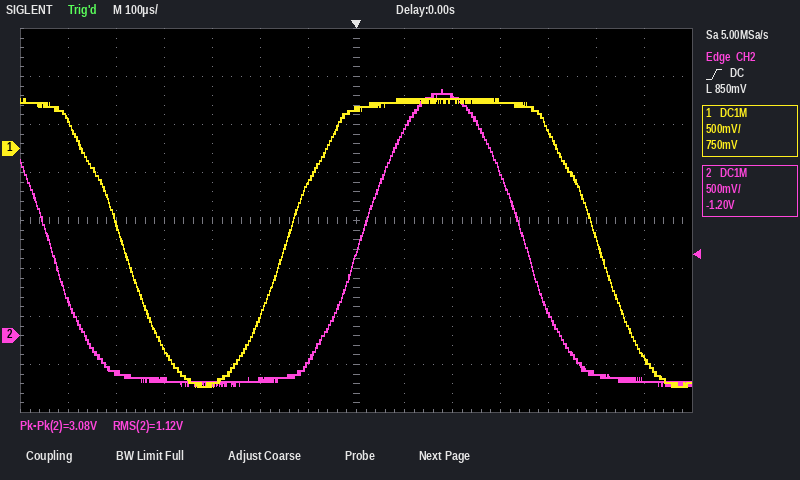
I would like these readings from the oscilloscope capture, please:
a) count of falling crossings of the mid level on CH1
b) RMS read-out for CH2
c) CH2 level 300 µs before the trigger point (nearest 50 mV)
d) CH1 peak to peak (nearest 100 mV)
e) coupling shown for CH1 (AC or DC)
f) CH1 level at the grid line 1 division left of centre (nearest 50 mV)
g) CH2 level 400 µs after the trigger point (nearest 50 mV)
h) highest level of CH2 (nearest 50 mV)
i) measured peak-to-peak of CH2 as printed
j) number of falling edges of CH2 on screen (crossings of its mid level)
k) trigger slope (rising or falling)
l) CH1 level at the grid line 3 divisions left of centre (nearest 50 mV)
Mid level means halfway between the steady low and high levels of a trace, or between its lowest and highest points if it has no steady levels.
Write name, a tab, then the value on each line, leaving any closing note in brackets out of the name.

count of falling crossings of the mid level on CH1	2
RMS read-out for CH2	1.12 V
CH2 level 300 µs before the trigger point	-500 mV
CH1 peak to peak	3.00 V
coupling shown for CH1	DC
CH1 level at the grid line 1 division left of centre	-350 mV
CH2 level 400 µs after the trigger point	250 mV
highest level of CH2	2.55 V
measured peak-to-peak of CH2 as printed	3.08 V
number of falling edges of CH2 on screen	2
trigger slope	rising
CH1 level at the grid line 3 divisions left of centre	-2.45 V
